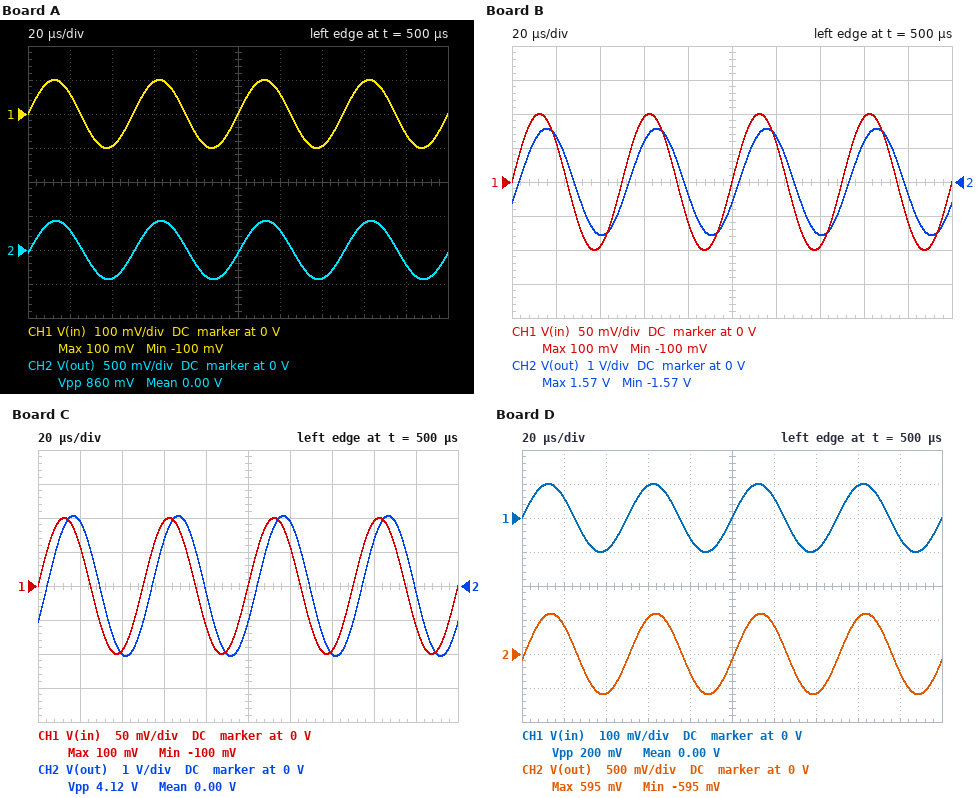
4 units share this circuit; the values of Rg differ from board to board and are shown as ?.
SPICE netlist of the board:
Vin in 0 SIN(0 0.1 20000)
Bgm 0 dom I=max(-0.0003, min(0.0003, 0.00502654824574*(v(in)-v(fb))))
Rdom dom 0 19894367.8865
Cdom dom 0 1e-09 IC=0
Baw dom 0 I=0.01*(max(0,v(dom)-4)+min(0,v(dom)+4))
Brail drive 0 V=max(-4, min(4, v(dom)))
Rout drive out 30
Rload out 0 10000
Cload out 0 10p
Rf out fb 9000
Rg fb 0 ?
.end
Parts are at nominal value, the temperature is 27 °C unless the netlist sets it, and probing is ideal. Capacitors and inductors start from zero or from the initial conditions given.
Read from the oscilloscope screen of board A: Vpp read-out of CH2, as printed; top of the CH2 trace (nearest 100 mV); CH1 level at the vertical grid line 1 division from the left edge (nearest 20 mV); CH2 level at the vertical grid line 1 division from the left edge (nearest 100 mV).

860 mV
400 mV
60 mV
300 mV
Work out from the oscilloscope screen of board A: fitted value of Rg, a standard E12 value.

2.7 kΩ
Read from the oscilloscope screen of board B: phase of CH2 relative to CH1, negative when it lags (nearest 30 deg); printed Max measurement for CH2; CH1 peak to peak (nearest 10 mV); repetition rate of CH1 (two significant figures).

-30 deg
1.57 V
200 mV
20 kHz
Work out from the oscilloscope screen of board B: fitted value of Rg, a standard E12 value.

560 Ω
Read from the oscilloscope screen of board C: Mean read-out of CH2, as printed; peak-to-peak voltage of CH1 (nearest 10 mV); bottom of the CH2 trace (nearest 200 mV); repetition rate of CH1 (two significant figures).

0.00 V
200 mV
-2.0 V
20 kHz
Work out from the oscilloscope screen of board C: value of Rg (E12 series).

390 Ω
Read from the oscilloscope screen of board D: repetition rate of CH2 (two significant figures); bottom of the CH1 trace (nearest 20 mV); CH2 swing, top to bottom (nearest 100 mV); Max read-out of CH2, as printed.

20 kHz
-100 mV
1.2 V
595 mV
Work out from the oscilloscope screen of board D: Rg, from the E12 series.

1.8 kΩ
